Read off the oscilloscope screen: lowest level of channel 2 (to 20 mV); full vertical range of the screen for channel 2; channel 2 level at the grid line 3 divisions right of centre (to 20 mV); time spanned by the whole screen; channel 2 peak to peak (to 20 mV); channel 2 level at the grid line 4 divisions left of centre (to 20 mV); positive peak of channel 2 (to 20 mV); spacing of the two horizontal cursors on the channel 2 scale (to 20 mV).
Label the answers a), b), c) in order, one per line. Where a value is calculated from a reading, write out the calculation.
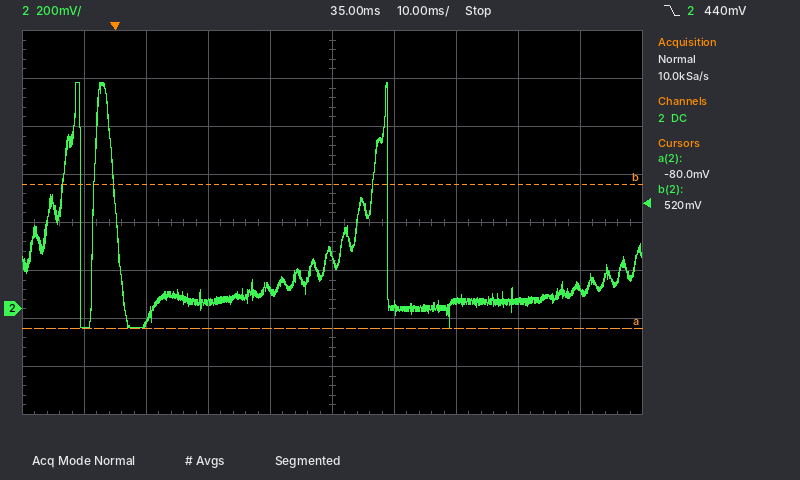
a) -80 mV
b) 1.6 V
c) 40 mV
d) 100 ms
e) 940 mV − (-80 mV) = 1.02 V
f) -80 mV
g) 940 mV
h) 600 mV
